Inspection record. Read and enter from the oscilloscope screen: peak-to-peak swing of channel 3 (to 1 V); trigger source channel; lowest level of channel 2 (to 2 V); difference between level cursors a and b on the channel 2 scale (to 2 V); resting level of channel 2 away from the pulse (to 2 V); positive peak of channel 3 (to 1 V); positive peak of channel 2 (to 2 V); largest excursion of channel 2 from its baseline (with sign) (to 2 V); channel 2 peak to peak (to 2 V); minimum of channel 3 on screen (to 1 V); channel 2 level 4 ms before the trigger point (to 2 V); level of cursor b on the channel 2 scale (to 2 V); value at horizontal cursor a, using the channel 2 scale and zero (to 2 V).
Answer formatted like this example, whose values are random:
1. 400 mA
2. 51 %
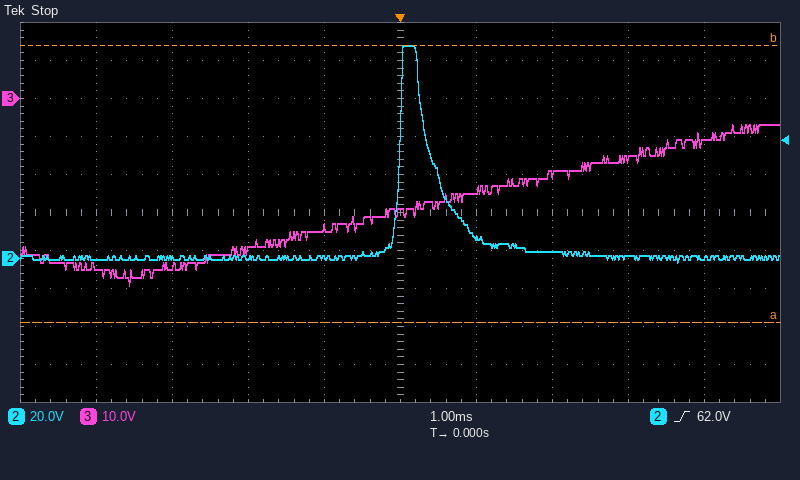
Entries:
1. 42 V
2. channel 2
3. -2 V
4. 146 V
5. 0 V
6. -7 V
7. 112 V
8. +112 V
9. 114 V
10. -49 V
11. 0 V
12. 112 V
13. -34 V
